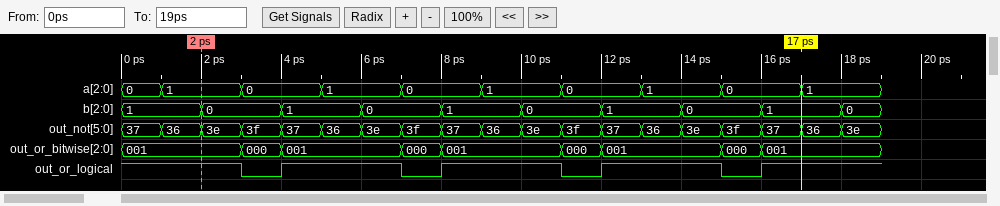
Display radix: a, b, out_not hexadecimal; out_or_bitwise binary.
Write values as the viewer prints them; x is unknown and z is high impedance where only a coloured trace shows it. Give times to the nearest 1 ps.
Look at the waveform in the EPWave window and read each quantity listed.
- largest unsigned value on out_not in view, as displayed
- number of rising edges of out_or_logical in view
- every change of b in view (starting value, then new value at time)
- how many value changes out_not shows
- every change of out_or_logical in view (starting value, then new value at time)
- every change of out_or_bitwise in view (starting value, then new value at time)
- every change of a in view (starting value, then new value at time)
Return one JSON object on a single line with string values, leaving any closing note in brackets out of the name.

{"largest unsigned value on out_not in view, as displayed": "3f", "number of rising edges of out_or_logical in view": "4", "every change of b in view": "1, 0 at 2 ps, 1 at 4 ps, 0 at 6 ps, 1 at 8 ps, 0 at 10 ps, 1 at 12 ps, 0 at 14 ps, 1 at 16 ps, 0 at 18 ps", "how many value changes out_not shows": "18", "every change of out_or_logical in view": "1, 0 at 3 ps, 1 at 4 ps, 0 at 7 ps, 1 at 8 ps, 0 at 11 ps, 1 at 12 ps, 0 at 15 ps, 1 at 16 ps", "every change of out_or_bitwise in view": "001, 000 at 3 ps, 001 at 4 ps, 000 at 7 ps, 001 at 8 ps, 000 at 11 ps, 001 at 12 ps, 000 at 15 ps, 001 at 16 ps", "every change of a in view": "0, 1 at 1 ps, 0 at 3 ps, 1 at 5 ps, 0 at 7 ps, 1 at 9 ps, 0 at 11 ps, 1 at 13 ps, 0 at 15 ps, 1 at 17 ps"}
